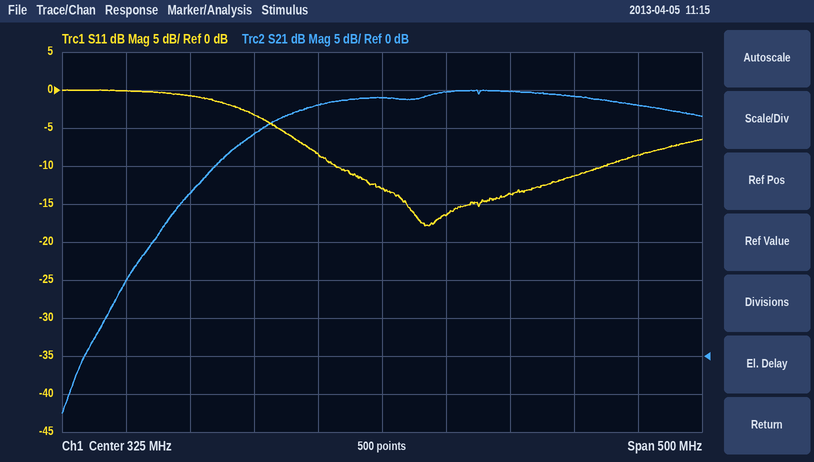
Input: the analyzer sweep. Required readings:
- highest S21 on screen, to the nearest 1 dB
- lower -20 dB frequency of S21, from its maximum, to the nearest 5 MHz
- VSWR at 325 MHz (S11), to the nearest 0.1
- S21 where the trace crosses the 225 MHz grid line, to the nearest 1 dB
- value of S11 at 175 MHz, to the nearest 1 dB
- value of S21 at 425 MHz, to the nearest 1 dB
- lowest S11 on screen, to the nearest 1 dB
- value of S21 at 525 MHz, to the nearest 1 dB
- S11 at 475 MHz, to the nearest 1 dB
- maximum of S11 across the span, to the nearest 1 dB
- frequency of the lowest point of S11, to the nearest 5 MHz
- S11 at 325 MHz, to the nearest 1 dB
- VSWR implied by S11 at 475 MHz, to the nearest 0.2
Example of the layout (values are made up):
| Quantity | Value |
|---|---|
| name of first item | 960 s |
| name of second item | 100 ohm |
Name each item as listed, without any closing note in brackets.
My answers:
| Quantity | Value |
|---|---|
| highest S21 on screen, to the nearest 1 dB | 35 dB |
| lower -20 dB frequency of S21, from its maximum, to the nearest 5 MHz | 145 MHz |
| VSWR at 325 MHz (S11), to the nearest 0.1 | 1.6 |
| S21 where the trace crosses the 225 MHz grid line, to the nearest 1 dB | 29 dB |
| value of S11 at 175 MHz, to the nearest 1 dB | -1 dB |
| value of S21 at 425 MHz, to the nearest 1 dB | 35 dB |
| lowest S11 on screen, to the nearest 1 dB | -18 dB |
| value of S21 at 525 MHz, to the nearest 1 dB | 33 dB |
| S11 at 475 MHz, to the nearest 1 dB | -11 dB |
| maximum of S11 across the span, to the nearest 1 dB | 0 dB |
| frequency of the lowest point of S11, to the nearest 5 MHz | 360 MHz |
| S11 at 325 MHz, to the nearest 1 dB | -13 dB |
| VSWR implied by S11 at 475 MHz, to the nearest 0.2 | 1.8 |
